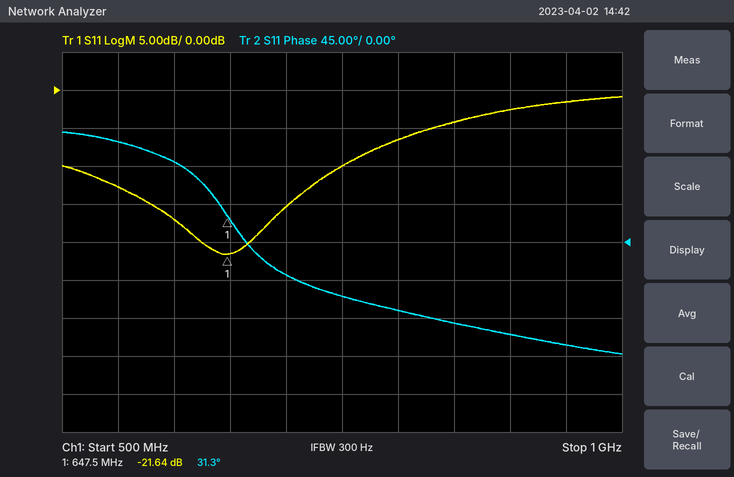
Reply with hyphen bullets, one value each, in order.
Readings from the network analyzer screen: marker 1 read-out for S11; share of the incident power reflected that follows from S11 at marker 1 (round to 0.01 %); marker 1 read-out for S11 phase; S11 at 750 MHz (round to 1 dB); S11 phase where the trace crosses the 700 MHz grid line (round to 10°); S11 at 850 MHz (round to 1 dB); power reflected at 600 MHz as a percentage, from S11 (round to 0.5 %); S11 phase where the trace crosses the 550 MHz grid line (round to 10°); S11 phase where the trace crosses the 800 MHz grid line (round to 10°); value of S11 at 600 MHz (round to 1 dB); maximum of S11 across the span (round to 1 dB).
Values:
- -21.64 dB
- 0.69 %
- 31.3°
- -10 dB
- -40°
- -4 dB
- 2.0 %
- 120°
- -80°
- -17 dB
- -1 dB
